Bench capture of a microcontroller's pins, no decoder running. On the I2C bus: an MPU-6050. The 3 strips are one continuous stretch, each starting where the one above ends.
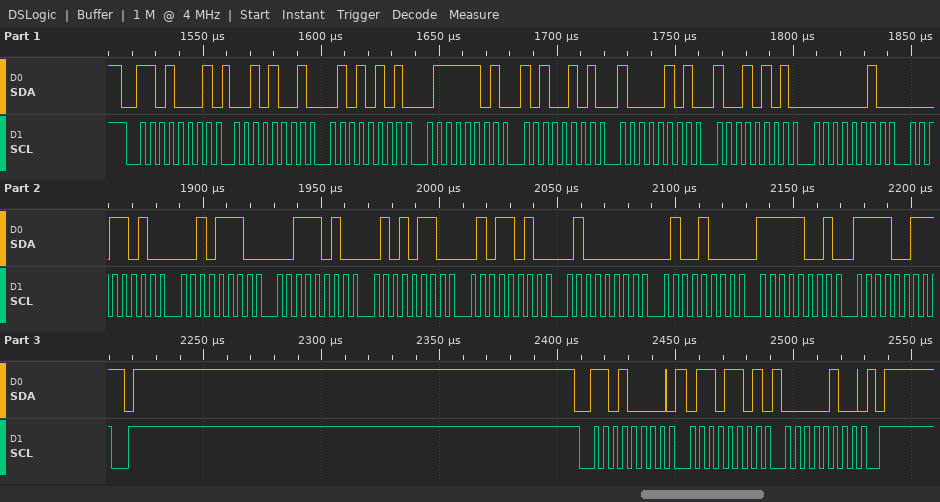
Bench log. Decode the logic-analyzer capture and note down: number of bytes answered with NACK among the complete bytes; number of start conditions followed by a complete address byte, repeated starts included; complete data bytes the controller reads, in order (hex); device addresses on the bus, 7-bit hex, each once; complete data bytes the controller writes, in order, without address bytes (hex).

1
2
29 55 7D A5 85 95 02 1A 2E 3A 56 5A 40 48 F9 F3
0x68
6D 04
